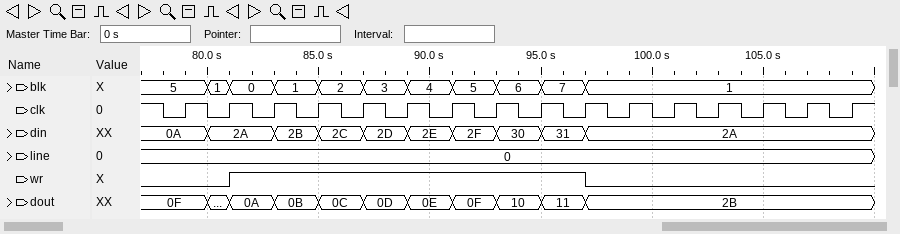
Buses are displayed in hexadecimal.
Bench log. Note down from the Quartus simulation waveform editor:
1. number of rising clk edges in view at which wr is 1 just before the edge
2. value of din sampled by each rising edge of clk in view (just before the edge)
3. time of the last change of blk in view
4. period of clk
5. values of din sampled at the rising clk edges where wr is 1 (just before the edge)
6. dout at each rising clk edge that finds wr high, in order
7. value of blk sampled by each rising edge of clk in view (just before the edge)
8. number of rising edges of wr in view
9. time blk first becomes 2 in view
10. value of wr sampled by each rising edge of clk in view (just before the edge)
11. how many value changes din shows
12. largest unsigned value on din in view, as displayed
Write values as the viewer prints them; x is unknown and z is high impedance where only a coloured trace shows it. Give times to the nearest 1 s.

8
0A, 2A, 2A, 2B, 2C, 2D, 2E, 2F, 30, 31, 2A, 2A, 2A, 2A, 2A, 2A
97 s
2 s
2A, 2B, 2C, 2D, 2E, 2F, 30, 31
0A, 0B, 0C, 0D, 0E, 0F, 10, 11
5, 1, 0, 1, 2, 3, 4, 5, 6, 7, 1, 1, 1, 1, 1, 1
1
85 s
0 0 1 1 1 1 1 1 1 1 0 0 0 0 0 0
9
31
